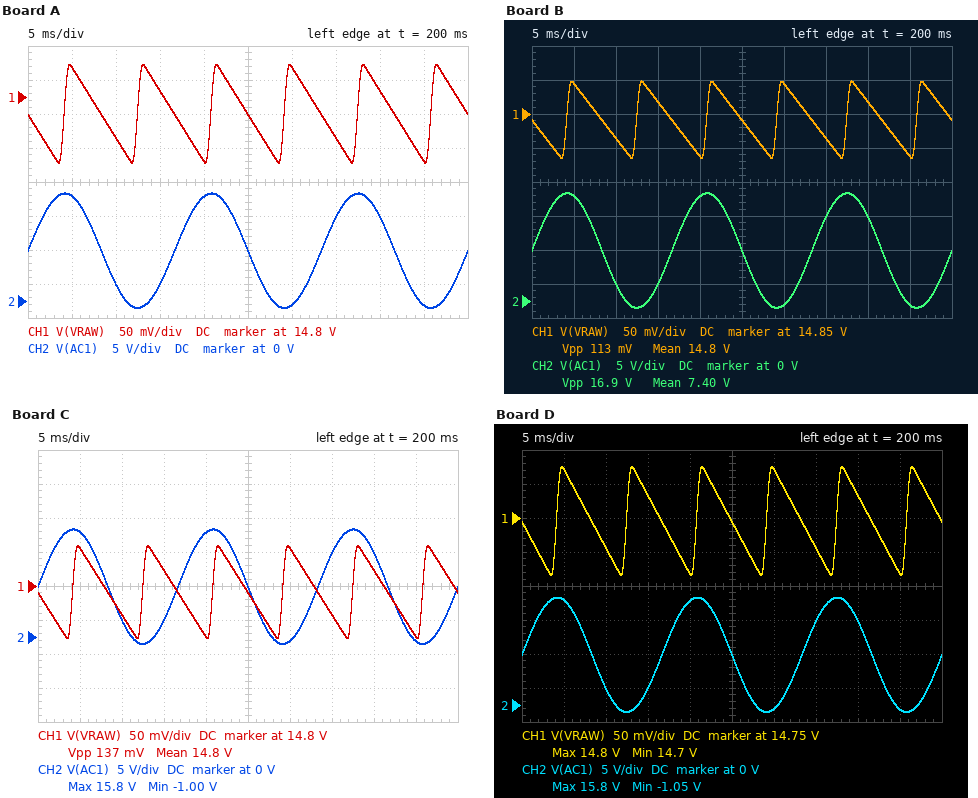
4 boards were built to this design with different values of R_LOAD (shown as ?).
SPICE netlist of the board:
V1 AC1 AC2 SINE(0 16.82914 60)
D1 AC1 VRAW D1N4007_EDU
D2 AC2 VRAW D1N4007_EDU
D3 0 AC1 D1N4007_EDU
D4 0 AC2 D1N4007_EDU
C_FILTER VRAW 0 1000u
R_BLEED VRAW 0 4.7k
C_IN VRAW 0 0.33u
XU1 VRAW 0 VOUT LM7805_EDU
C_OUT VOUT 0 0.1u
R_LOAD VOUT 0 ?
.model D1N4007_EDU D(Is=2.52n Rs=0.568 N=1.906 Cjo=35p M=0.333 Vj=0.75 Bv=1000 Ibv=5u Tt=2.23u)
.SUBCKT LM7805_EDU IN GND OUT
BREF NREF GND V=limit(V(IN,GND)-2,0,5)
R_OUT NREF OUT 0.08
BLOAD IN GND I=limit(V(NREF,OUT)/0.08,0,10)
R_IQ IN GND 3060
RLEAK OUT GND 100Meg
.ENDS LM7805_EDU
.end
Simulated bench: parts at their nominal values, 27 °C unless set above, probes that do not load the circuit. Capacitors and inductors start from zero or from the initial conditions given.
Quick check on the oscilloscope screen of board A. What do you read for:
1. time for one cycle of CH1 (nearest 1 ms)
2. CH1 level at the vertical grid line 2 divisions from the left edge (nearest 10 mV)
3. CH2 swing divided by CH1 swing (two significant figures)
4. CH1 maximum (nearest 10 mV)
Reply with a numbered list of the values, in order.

1. 8 ms
2. 14.74 V
3. 120
4. 14.85 V
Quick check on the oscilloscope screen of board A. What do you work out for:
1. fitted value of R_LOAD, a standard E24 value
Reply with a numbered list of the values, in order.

1. 390 Ω
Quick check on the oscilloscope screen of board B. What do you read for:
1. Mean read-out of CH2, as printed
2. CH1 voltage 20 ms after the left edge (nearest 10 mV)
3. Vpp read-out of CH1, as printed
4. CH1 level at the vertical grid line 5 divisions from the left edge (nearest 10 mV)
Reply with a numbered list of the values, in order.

1. 7.40 V
2. 14.79 V
3. 113 mV
4. 14.84 V
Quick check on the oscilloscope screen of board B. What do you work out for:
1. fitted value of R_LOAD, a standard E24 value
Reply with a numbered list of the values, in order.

1. 620 Ω
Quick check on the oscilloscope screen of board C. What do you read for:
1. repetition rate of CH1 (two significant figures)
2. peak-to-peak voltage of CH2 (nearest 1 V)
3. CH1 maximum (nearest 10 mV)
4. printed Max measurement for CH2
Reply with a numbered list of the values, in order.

1. 120 Hz
2. 17 V
3. 14.86 V
4. 15.8 V
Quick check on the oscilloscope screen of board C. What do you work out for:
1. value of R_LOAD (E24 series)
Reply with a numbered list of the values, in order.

1. 430 Ω
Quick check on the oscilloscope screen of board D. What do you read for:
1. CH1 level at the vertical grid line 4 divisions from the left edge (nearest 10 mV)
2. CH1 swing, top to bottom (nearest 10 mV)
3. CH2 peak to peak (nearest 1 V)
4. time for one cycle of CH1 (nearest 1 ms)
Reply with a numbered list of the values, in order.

1. 14.67 V
2. 160 mV
3. 17 V
4. 8 ms
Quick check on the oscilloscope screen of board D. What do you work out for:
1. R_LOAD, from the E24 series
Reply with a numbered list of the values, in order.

1. 330 Ω
